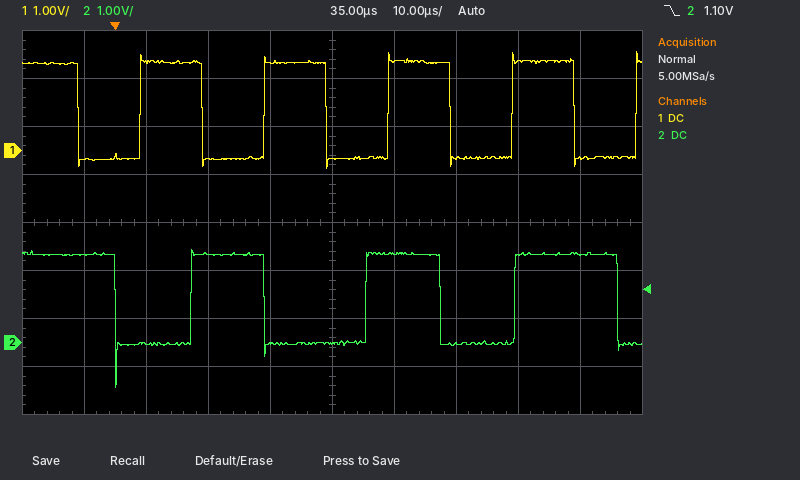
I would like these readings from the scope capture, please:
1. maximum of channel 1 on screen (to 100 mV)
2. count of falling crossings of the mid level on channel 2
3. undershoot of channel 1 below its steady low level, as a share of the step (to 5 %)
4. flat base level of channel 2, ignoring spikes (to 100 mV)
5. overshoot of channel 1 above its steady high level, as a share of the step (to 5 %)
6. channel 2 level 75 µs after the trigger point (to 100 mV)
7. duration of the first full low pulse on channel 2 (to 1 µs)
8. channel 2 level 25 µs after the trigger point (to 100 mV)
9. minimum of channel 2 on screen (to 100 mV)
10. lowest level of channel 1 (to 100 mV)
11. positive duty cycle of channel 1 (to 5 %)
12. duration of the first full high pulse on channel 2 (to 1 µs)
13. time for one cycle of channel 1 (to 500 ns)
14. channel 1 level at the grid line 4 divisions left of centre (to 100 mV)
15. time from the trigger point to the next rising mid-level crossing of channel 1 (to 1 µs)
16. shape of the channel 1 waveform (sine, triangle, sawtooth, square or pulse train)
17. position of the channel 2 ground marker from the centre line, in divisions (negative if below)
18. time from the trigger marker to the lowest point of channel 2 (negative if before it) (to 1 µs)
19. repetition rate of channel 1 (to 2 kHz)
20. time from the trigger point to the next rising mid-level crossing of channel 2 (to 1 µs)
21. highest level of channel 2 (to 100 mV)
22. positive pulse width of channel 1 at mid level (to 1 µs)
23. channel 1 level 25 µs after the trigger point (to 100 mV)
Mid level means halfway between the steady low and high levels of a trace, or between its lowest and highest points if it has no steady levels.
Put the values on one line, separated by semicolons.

2.1 V; 4; 10 %; 0.0 V; 10 %; 1.8 V; 12 µs; 0.0 V; -900 mV; -400 mV; 50 %; 12 µs; 20.0 µs; -200 mV; 4 µs; square; -2.5 div; 0 µs; 50 kHz; 12 µs; 1.9 V; 10 µs; 1.8 V
